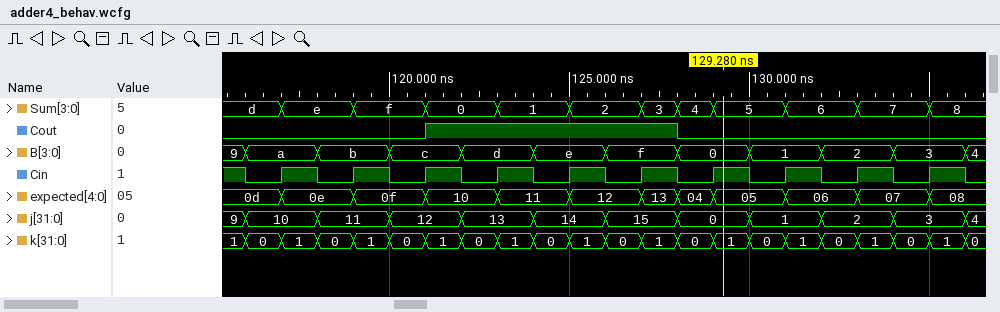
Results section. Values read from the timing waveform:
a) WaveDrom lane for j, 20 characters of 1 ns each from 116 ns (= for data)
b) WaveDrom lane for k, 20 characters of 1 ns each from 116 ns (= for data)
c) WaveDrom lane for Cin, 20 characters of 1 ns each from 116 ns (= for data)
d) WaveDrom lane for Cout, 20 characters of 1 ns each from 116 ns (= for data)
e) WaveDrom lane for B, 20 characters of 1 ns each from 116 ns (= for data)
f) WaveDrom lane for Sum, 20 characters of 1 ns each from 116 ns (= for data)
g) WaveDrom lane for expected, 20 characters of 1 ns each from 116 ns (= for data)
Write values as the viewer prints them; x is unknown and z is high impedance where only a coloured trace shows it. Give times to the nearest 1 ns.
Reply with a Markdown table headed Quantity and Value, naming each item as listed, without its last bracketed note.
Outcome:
| Quantity | Value |
|---|---|
| WaveDrom lane for j, 20 characters of 1 ns each from 116 ns | {name: 'j', wave: '=.=.=.=.=.=.=.=.=.=.', data: '10 11 12 13 14 15 0 1 2 3'} |
| WaveDrom lane for k, 20 characters of 1 ns each from 116 ns | {name: 'k', wave: '====================', data: '0 1 0 1 0 1 0 1 0 1 0 1 0 1 0 1 0 1 0 1'} |
| WaveDrom lane for Cin, 20 characters of 1 ns each from 116 ns | {name: 'Cin', wave: '01010101010101010101'} |
| WaveDrom lane for Cout, 20 characters of 1 ns each from 116 ns | {name: 'Cout', wave: '0....1......0.......'} |
| WaveDrom lane for B, 20 characters of 1 ns each from 116 ns | {name: 'B', wave: '=.=.=.=.=.=.=.=.=.=.', data: 'a b c d e f 0 1 2 3'} |
| WaveDrom lane for Sum, 20 characters of 1 ns each from 116 ns | {name: 'Sum', wave: '==.=.=.=.=.===.=.=.=', data: 'd e f 0 1 2 3 4 5 6 7 8'} |
| WaveDrom lane for expected, 20 characters of 1 ns each from 116 ns | {name: 'expected', wave: '==.=.=.=.=.===.=.=.=', data: '0d 0e 0f 10 11 12 13 04 05 06 07 08'} |
